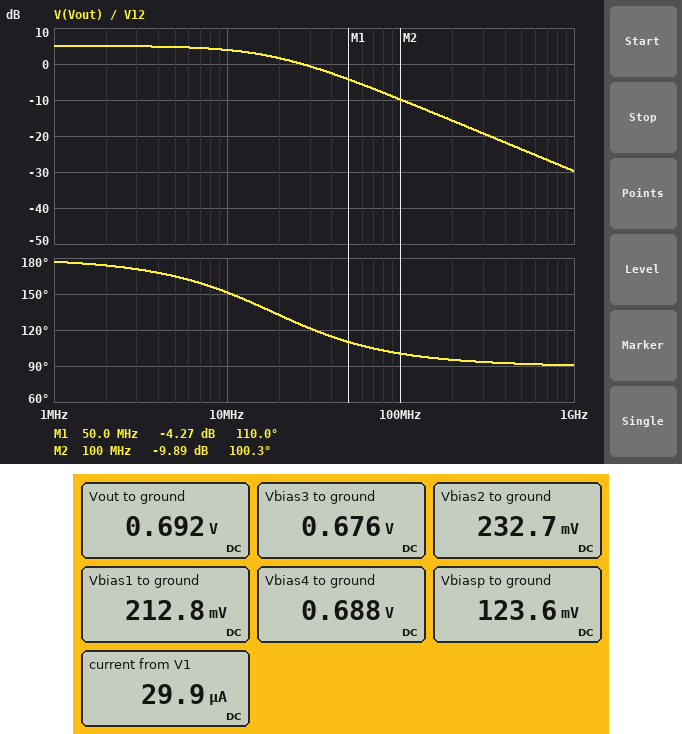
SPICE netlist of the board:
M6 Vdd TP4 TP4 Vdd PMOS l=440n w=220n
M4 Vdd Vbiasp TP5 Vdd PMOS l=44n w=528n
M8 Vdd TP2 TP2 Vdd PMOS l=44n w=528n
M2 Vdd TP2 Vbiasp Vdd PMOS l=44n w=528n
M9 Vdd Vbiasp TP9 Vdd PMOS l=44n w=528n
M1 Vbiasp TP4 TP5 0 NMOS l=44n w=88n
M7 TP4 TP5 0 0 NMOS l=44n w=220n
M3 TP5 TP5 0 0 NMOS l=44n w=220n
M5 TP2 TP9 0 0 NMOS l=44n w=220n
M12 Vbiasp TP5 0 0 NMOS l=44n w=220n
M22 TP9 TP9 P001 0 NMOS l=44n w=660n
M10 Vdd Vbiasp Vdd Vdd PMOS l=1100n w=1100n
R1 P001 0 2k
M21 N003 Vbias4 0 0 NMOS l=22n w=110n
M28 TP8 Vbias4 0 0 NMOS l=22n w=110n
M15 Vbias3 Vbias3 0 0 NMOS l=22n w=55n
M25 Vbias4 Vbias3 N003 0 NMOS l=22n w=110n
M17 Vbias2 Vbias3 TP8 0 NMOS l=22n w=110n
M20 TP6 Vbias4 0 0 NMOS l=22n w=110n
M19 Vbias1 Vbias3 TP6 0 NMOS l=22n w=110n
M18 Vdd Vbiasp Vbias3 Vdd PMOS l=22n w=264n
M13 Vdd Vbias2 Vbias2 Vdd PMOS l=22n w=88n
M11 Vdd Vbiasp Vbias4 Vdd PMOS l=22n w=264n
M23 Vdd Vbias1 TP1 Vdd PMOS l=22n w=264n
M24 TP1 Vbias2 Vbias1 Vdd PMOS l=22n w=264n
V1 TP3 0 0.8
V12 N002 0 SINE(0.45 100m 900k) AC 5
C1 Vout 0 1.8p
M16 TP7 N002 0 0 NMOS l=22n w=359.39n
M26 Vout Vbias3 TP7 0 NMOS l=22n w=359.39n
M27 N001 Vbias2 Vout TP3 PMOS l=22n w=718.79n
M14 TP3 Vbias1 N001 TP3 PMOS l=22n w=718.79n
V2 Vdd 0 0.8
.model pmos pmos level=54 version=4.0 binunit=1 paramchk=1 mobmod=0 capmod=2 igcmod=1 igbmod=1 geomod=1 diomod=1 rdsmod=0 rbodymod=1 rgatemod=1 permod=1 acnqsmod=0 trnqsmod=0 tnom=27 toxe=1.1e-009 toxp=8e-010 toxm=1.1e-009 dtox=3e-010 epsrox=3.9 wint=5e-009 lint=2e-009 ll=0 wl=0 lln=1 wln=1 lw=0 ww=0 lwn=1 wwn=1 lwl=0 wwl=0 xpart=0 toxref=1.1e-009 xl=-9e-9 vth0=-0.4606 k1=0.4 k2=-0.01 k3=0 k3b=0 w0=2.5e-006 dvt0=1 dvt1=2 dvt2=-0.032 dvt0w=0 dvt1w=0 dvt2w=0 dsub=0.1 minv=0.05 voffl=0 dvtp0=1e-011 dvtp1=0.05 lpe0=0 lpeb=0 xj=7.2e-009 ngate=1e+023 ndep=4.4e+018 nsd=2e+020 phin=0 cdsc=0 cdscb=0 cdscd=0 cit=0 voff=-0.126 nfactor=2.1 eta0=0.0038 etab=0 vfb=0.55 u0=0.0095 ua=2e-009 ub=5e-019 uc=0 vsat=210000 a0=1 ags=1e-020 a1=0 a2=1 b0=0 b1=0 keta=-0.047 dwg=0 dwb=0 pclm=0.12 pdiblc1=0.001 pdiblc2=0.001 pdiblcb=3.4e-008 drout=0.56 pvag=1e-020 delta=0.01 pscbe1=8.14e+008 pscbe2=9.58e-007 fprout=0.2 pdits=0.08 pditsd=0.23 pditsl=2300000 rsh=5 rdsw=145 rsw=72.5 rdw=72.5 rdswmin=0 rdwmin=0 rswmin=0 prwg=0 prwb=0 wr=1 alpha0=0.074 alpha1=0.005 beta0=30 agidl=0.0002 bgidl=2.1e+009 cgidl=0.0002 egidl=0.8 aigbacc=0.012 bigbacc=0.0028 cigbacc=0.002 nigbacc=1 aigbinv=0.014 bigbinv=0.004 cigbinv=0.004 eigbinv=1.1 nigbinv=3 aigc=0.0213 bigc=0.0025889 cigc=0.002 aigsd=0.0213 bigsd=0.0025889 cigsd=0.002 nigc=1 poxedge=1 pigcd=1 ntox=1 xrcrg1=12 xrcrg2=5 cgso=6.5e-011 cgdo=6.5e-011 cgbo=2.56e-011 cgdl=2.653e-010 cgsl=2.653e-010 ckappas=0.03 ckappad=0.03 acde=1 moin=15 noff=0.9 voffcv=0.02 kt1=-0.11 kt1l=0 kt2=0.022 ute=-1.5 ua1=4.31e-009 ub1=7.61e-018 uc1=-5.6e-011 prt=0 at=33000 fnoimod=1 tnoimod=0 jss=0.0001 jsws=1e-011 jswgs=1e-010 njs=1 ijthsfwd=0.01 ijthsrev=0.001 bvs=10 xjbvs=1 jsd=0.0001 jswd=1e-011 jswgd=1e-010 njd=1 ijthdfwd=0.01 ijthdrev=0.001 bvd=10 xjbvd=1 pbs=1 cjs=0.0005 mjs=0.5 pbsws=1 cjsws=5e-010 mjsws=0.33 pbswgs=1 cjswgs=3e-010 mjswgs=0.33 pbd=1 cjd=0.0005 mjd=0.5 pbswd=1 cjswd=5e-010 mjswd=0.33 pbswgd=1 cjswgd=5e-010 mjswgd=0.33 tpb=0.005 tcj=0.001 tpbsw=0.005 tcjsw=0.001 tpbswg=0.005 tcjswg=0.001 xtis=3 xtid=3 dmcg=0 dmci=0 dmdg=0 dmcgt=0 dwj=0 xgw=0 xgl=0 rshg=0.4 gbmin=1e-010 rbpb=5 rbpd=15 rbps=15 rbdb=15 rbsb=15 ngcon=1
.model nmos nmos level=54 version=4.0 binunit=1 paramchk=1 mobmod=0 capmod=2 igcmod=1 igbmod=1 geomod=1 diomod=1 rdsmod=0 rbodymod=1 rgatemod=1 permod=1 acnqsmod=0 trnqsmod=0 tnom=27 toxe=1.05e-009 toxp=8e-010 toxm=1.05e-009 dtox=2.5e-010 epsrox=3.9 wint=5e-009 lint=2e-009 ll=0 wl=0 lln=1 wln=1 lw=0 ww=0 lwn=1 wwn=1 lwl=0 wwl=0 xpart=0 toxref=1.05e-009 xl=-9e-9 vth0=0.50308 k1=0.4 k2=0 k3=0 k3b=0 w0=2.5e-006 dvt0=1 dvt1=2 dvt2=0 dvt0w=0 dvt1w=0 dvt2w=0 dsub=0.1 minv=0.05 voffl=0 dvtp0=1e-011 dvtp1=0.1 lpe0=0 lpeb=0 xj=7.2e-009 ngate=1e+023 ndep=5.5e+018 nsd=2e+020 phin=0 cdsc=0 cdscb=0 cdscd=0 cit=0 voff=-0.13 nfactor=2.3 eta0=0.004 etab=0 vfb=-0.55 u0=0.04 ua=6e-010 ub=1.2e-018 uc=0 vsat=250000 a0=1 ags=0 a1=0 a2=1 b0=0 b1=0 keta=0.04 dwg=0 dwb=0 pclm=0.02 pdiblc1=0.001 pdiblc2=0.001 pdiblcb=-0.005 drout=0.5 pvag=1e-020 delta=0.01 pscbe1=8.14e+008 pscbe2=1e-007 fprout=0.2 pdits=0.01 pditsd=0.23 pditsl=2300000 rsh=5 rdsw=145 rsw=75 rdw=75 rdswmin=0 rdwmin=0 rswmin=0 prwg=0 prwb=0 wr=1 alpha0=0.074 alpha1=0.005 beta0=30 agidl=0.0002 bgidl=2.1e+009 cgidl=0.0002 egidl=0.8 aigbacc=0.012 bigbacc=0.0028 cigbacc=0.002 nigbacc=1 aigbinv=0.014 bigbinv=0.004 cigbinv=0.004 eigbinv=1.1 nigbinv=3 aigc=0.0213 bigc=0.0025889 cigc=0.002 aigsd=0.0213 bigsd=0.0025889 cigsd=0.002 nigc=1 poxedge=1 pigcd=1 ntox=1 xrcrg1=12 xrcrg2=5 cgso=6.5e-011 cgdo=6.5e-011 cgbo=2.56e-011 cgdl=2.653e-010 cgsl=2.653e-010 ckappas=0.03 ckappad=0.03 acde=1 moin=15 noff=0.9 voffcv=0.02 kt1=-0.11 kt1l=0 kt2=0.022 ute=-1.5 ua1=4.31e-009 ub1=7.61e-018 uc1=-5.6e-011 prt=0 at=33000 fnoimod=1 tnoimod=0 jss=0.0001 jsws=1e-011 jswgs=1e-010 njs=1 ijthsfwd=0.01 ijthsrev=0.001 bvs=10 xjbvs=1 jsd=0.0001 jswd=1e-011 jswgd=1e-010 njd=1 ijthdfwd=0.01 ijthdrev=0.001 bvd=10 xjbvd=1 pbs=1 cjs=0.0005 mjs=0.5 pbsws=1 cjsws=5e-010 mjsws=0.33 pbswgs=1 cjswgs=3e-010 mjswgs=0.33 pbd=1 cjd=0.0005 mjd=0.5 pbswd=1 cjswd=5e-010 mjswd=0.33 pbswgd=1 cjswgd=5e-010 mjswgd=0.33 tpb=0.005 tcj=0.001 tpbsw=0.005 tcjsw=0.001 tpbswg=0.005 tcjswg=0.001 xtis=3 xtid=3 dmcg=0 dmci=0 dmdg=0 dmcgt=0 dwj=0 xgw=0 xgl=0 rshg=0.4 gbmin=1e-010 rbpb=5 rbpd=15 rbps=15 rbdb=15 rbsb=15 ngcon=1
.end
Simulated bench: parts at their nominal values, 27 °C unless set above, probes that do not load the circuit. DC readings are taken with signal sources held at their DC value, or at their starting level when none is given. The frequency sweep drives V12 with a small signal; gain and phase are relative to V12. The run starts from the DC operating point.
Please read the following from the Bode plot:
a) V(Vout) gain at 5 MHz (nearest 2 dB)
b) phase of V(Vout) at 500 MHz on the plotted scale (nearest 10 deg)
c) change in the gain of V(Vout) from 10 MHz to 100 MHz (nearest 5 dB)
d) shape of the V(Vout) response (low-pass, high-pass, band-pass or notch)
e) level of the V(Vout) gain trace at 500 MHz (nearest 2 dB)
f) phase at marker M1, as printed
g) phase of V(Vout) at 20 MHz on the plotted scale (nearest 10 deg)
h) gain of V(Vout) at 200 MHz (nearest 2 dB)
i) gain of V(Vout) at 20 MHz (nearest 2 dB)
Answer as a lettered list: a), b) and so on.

a) 4 dB
b) 90 deg
c) -15 dB
d) low-pass
e) -24 dB
f) 110.0 deg
g) 130 deg
h) -16 dB
i) 2 dB
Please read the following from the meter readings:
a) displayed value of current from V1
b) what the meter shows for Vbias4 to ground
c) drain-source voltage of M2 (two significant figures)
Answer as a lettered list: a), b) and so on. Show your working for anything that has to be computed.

a) 29.9 µA
b) 0.688 V
c) 800 mV - 123.6 mV = 680 mV
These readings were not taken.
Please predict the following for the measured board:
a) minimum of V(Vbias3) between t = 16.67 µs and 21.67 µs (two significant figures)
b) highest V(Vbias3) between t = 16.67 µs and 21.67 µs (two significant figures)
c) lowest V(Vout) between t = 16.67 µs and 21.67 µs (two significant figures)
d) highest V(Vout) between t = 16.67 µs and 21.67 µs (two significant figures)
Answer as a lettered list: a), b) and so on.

a) 680 mV
b) 680 mV
c) 320 mV
d) 780 mV
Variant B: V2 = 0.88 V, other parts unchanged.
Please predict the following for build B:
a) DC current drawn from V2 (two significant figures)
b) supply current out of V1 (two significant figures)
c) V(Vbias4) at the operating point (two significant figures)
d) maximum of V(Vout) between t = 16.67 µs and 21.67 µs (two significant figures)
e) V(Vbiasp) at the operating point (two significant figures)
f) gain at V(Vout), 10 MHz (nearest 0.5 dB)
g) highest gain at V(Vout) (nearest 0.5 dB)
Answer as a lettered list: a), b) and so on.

a) 330 µA
b) 32 µA
c) 740 mV
d) 770 mV
e) 180 mV
f) 9.0 dB
g) 13.5 dB
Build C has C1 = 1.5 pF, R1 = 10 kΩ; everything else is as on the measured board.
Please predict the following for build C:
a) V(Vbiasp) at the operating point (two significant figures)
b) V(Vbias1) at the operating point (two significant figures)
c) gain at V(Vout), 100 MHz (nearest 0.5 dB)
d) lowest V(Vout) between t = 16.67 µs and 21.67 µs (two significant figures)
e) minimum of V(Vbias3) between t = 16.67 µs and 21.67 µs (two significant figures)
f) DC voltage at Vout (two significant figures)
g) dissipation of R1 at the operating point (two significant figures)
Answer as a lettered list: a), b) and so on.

a) 300 mV
b) 270 mV
c) -10.5 dB
d) 250 mV
e) 560 mV
f) 610 mV
g) 220 nW
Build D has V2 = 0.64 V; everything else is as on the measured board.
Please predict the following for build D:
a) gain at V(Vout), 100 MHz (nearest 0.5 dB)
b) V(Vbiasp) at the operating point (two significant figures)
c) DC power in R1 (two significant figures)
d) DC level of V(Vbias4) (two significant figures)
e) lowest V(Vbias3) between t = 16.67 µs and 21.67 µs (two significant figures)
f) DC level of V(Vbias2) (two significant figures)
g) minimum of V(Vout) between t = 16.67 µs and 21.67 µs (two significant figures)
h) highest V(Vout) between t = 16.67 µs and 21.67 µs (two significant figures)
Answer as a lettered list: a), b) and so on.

a) -12.0 dB
b) 50 mV
c) 320 nW
d) 570 mV
e) 550 mV
f) 170 mV
g) 640 mV
h) 790 mV
